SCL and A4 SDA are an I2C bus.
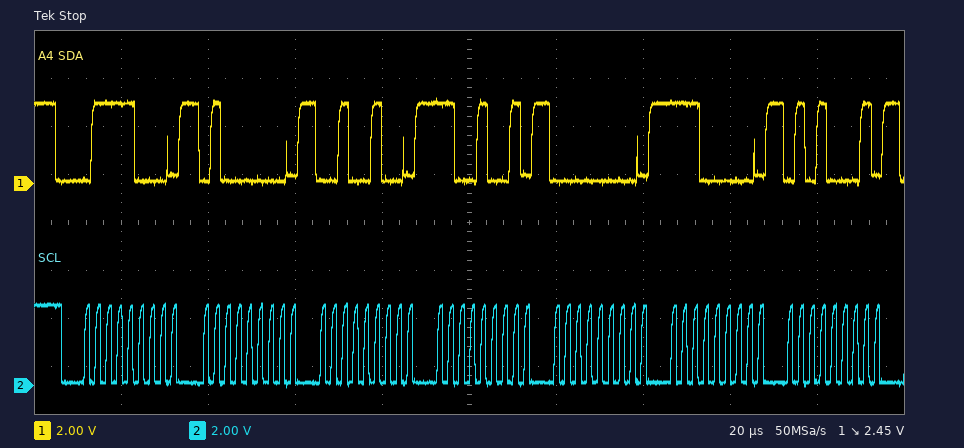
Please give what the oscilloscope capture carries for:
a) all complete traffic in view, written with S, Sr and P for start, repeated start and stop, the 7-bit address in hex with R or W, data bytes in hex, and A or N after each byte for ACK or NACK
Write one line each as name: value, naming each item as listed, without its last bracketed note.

all complete traffic in view, written with S, Sr and P for start, repeated start and stop, the 7-bit address in hex with R or W, data bytes in hex, and A or N after each byte for ACK or NACK: S 3CW A 40 A 24 A C9 A 00 A E0 A 51 A
